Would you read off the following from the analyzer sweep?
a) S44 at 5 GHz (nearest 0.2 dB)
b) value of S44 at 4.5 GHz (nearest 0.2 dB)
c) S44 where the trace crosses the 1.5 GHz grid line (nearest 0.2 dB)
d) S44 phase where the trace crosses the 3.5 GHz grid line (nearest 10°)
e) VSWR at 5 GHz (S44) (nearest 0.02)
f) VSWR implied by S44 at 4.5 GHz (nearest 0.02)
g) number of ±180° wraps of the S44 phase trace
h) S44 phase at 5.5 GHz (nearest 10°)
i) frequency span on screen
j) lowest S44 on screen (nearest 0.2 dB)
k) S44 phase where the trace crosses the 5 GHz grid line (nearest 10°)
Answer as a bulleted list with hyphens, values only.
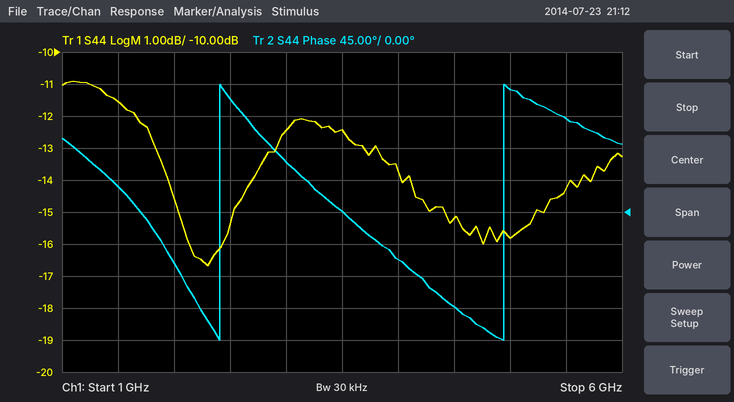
- -15.8 dB
- -15.2 dB
- -11.6 dB
- 0°
- 1.38
- 1.42
- 2
- 130°
- 5 GHz
- -16.6 dB
- 170°
